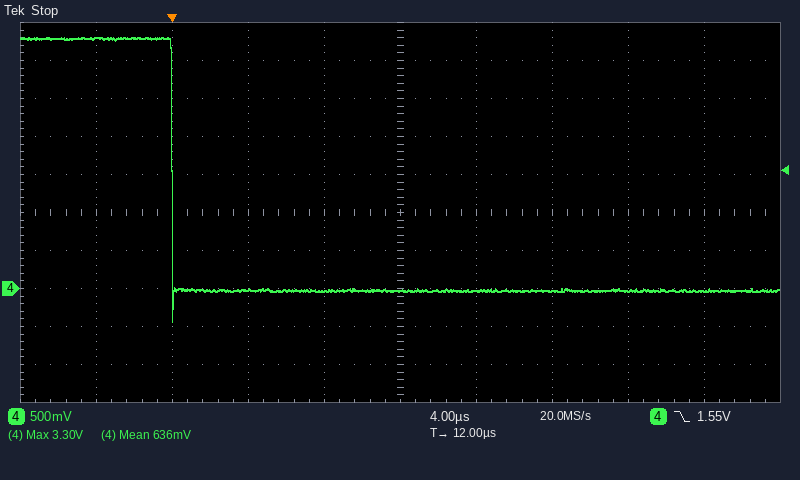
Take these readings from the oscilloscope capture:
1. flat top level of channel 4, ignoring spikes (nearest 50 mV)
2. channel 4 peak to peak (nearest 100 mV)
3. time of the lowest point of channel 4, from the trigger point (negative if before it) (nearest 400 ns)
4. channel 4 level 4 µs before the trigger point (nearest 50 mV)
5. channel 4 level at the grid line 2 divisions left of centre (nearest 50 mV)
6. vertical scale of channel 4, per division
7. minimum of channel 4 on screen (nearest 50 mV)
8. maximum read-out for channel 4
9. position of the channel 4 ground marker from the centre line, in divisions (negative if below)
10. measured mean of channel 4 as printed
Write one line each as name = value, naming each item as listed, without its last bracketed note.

flat top level of channel 4, ignoring spikes = 3.30 V
channel 4 peak to peak = 3.70 V
time of the lowest point of channel 4, from the trigger point (negative if before it) = 0.0 µs
channel 4 level 4 µs before the trigger point = 3.30 V
channel 4 level at the grid line 2 divisions left of centre = 0 mV
vertical scale of channel 4, per division = 500 mV
minimum of channel 4 on screen = -450 mV
maximum read-out for channel 4 = 3.30 V
position of the channel 4 ground marker from the centre line, in divisions = -2.0 div
measured mean of channel 4 as printed = 636 mV
